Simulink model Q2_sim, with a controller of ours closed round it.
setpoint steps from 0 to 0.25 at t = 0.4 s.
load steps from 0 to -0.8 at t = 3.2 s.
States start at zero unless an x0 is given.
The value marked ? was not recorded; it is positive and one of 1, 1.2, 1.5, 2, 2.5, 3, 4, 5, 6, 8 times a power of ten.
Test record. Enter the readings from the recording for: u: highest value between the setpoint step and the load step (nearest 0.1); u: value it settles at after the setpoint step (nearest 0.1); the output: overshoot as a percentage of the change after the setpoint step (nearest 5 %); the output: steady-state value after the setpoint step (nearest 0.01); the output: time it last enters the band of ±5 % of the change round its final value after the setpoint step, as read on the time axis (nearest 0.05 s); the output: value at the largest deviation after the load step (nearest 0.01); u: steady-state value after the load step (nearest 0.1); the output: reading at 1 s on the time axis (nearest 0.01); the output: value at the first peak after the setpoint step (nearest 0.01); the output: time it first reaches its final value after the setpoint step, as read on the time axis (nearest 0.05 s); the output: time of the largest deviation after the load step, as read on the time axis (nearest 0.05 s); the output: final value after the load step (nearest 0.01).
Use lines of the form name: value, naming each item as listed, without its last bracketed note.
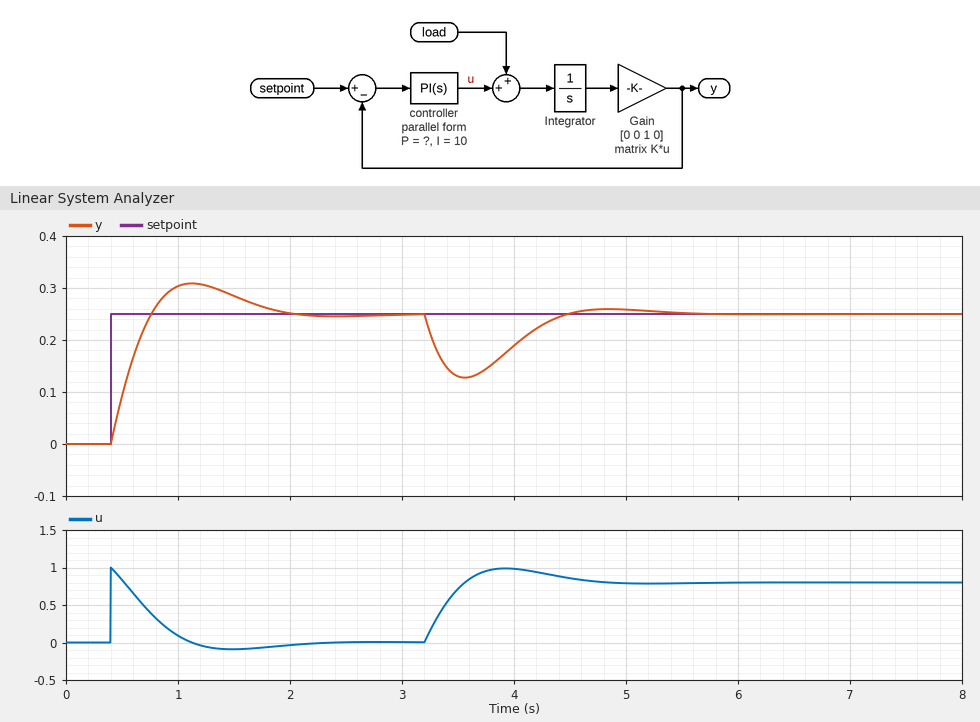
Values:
u: highest value between the setpoint step and the load step: 1.0
u: value it settles at after the setpoint step: 0.0
the output: overshoot as a percentage of the change after the setpoint step: 25 %
the output: steady-state value after the setpoint step: 0.25
the output: time it last enters the band of ±5 % of the change round its final value after the setpoint step, as read on the time axis: 1.80 s
the output: value at the largest deviation after the load step: 0.13
u: steady-state value after the load step: 0.8
the output: reading at 1 s on the time axis: 0.30
the output: value at the first peak after the setpoint step: 0.31
the output: time it first reaches its final value after the setpoint step, as read on the time axis: 0.75 s
the output: time of the largest deviation after the load step, as read on the time axis: 3.55 s
the output: final value after the load step: 0.25
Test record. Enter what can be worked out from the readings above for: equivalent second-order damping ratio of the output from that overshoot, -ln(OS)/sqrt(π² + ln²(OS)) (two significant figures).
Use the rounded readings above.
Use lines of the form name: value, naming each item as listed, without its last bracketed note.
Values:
equivalent second-order damping ratio of the output from that overshoot, -ln(OS)/sqrt(π² + ln²(OS)): 0.40
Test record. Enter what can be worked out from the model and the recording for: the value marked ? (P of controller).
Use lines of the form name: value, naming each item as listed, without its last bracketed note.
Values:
the value marked ?: 4
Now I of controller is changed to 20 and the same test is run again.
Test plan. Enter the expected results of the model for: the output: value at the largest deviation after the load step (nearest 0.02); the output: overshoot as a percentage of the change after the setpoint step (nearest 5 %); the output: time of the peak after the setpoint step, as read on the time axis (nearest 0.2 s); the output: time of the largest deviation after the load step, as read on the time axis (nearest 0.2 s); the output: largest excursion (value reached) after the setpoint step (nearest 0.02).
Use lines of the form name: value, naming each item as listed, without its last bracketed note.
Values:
the output: value at the largest deviation after the load step: 0.14
the output: overshoot as a percentage of the change after the setpoint step: 35 %
the output: time of the peak after the setpoint step, as read on the time axis: 1.0 s
the output: time of the largest deviation after the load step, as read on the time axis: 3.4 s
the output: largest excursion (value reached) after the setpoint step: 0.34
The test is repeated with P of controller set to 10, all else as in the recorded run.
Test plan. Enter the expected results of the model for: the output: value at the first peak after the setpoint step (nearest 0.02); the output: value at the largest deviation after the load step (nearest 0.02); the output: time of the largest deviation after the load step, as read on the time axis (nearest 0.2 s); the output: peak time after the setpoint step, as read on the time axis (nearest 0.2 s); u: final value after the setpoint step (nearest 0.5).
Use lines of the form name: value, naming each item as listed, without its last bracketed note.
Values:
the output: value at the first peak after the setpoint step: 0.26
the output: value at the largest deviation after the load step: 0.18
the output: time of the largest deviation after the load step, as read on the time axis: 3.4 s
the output: peak time after the setpoint step, as read on the time axis: 1.0 s
u: final value after the setpoint step: 0.0
